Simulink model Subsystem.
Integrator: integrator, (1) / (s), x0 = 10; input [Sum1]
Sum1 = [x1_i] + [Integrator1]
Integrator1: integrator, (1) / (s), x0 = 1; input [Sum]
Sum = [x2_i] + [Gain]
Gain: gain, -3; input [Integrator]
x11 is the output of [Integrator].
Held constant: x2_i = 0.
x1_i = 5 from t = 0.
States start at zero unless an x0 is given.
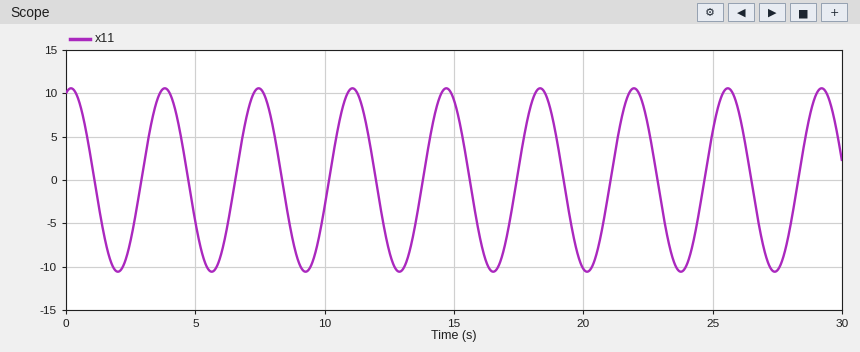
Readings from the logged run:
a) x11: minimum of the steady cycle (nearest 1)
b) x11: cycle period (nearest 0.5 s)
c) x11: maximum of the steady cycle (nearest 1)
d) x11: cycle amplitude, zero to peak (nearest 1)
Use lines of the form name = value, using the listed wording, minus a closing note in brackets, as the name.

x11: minimum of the steady cycle = -11
x11: cycle period = 3.5 s
x11: maximum of the steady cycle = 11
x11: cycle amplitude, zero to peak = 11
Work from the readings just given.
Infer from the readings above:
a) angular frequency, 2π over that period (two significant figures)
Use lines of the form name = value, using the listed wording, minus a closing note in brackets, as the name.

angular frequency, 2π over that period = 1.8 rad/s
